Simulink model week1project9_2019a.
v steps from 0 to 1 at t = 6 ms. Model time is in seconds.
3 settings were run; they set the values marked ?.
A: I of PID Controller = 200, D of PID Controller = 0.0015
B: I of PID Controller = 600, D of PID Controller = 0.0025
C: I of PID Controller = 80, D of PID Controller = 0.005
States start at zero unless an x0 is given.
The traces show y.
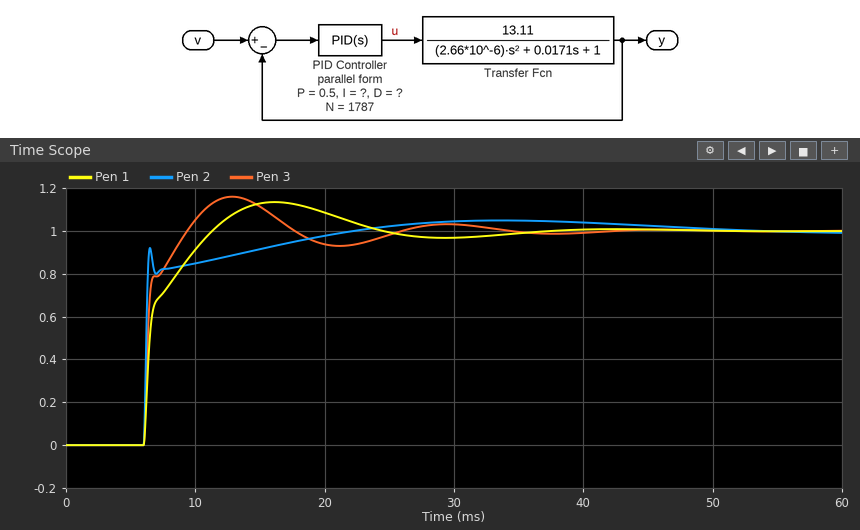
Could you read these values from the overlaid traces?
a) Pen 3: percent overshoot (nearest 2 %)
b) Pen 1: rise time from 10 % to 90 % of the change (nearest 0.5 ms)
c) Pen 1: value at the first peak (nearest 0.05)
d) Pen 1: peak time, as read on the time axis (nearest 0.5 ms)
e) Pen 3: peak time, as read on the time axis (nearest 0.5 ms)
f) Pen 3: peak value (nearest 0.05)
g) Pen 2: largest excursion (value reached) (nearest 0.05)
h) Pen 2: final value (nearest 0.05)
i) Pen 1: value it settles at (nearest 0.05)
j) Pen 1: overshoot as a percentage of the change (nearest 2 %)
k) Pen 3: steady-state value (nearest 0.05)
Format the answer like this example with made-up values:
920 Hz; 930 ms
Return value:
16 %; 3.5 ms; 1.15; 16.0 ms; 13.0 ms; 1.15; 1.05; 1.00; 1.00; 14 %; 1.00
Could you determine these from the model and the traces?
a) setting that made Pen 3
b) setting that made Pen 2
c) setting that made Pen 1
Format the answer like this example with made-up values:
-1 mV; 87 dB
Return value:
B; C; A
